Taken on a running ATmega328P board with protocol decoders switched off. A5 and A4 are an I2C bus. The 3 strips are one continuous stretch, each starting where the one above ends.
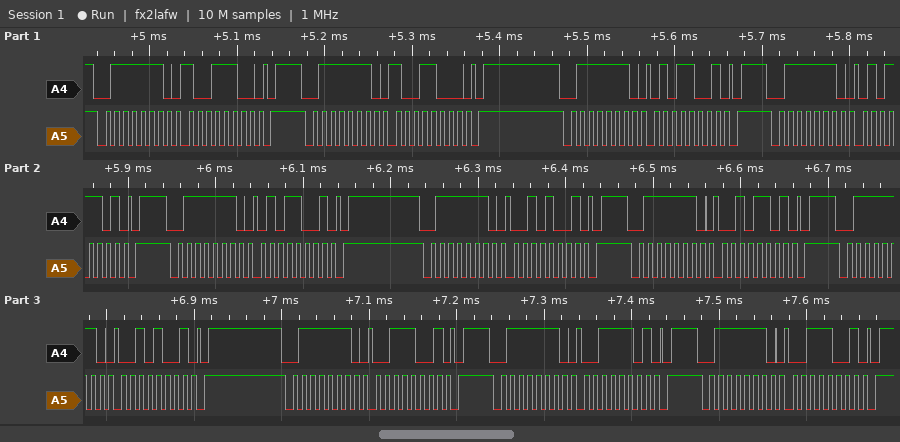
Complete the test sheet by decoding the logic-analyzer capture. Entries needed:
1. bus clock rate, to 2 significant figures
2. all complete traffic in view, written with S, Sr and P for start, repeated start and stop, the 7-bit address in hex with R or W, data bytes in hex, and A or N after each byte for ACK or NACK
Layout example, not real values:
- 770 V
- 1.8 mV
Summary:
- 100 kHz
- S 3FW A 9C A P S 3FW A 98 A P S 3FW A 59 A P S 3FW A 5D A P S 3FW A 59 A P S 3FW A 29 A P S 3FW A 2D A P S 3FW A 29 A P S 3FW A 39 A P S 3FW A 3D A P S 3FW A 39 A P
